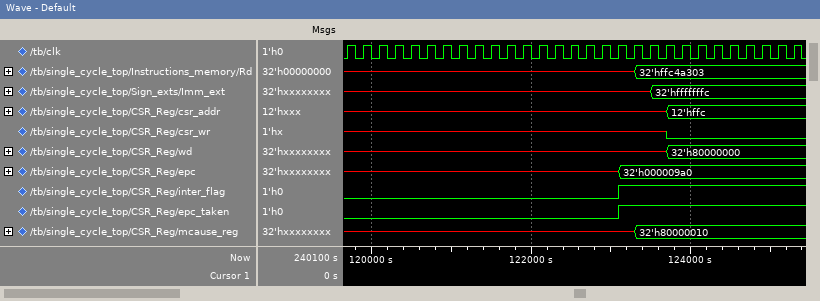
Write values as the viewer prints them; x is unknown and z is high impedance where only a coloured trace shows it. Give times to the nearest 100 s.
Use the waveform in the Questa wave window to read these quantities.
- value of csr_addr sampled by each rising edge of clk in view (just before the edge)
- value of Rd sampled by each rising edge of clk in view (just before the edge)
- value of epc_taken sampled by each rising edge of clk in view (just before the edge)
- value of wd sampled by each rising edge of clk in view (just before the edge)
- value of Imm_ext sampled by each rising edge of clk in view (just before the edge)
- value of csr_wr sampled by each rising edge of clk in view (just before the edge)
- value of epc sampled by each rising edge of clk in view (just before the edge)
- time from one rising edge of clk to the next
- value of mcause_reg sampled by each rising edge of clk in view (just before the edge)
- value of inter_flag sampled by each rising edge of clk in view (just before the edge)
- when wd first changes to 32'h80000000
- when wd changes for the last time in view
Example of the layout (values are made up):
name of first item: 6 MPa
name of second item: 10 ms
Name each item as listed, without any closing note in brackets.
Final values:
value of csr_addr sampled by each rising edge of clk in view: x, x, x, x, x, x, x, x, x, x, x, x, x, x, x, x, x, x, x, x, x, 12'hffc, 12'hffc, 12'hffc, 12'hffc, 12'hffc, 12'hffc, 12'hffc, 12'hffc
value of Rd sampled by each rising edge of clk in view: x, x, x, x, x, x, x, x, x, x, x, x, x, x, x, x, x, x, x, 32'hffc4a303, 32'hffc4a303, 32'hffc4a303, 32'hffc4a303, 32'hffc4a303, 32'hffc4a303, 32'hffc4a303, 32'hffc4a303, 32'hffc4a303, 32'hffc4a303
value of epc_taken sampled by each rising edge of clk in view: 0 0 0 0 0 0 0 0 0 0 0 0 0 0 0 0 0 0 1 1 1 1 1 1 1 1 1 1 1
value of wd sampled by each rising edge of clk in view: x, x, x, x, x, x, x, x, x, x, x, x, x, x, x, x, x, x, x, x, x, 32'h80000000, 32'h80000000, 32'h80000000, 32'h80000000, 32'h80000000, 32'h80000000, 32'h80000000, 32'h80000000
value of Imm_ext sampled by each rising edge of clk in view: x, x, x, x, x, x, x, x, x, x, x, x, x, x, x, x, x, x, x, x, 32'hfffffffc, 32'hfffffffc, 32'hfffffffc, 32'hfffffffc, 32'hfffffffc, 32'hfffffffc, 32'hfffffffc, 32'hfffffffc, 32'hfffffffc
value of csr_wr sampled by each rising edge of clk in view: x x x x x x x x x x x x x x x x x x x x x 0 0 0 0 0 0 0 0
value of epc sampled by each rising edge of clk in view: x, x, x, x, x, x, x, x, x, x, x, x, x, x, x, x, x, x, 32'h000009a0, 32'h000009a0, 32'h000009a0, 32'h000009a0, 32'h000009a0, 32'h000009a0, 32'h000009a0, 32'h000009a0, 32'h000009a0, 32'h000009a0, 32'h000009a0
time from one rising edge of clk to the next: 200 s
value of mcause_reg sampled by each rising edge of clk in view: x, x, x, x, x, x, x, x, x, x, x, x, x, x, x, x, x, x, x, 32'h80000010, 32'h80000010, 32'h80000010, 32'h80000010, 32'h80000010, 32'h80000010, 32'h80000010, 32'h80000010, 32'h80000010, 32'h80000010
value of inter_flag sampled by each rising edge of clk in view: 0 0 0 0 0 0 0 0 0 0 0 0 0 0 0 0 0 0 1 1 1 1 1 1 1 1 1 1 1
when wd first changes to 32'h80000000: 123700 s
when wd changes for the last time in view: 123700 s
